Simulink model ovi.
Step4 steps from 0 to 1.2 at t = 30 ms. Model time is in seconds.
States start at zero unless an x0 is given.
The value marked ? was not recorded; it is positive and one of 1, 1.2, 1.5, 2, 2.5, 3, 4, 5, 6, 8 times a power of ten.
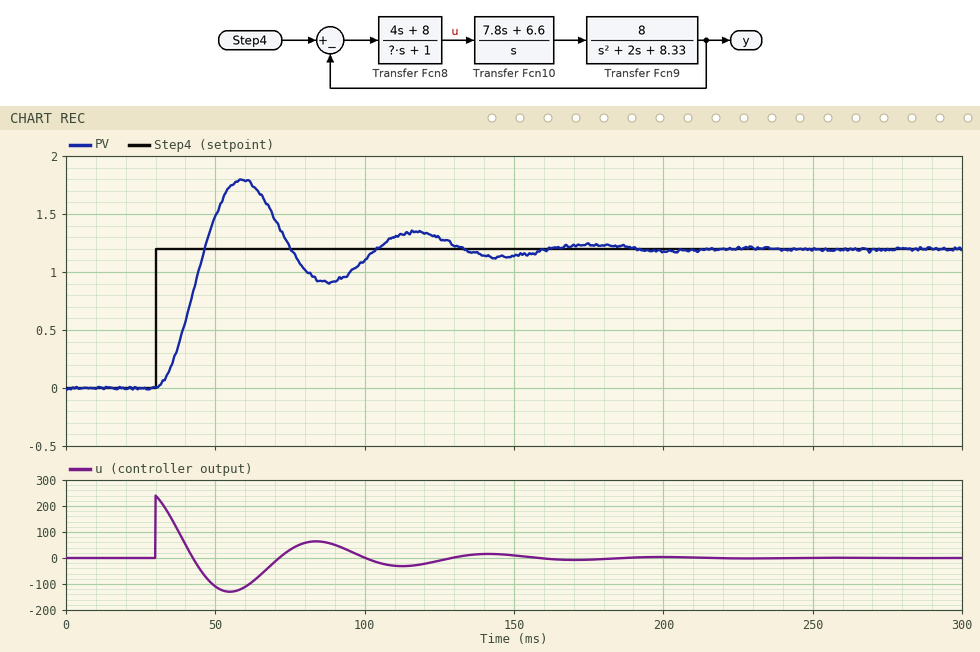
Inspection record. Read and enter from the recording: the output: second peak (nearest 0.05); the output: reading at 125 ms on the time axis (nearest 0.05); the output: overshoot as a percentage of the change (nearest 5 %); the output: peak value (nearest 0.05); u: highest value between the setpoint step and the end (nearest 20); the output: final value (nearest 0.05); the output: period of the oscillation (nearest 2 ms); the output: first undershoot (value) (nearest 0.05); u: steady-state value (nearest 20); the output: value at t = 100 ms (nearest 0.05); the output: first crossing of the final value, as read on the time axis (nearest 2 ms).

1.35
1.30
50 %
1.80
240
1.20
58 ms
0.90
0
1.10
46 ms
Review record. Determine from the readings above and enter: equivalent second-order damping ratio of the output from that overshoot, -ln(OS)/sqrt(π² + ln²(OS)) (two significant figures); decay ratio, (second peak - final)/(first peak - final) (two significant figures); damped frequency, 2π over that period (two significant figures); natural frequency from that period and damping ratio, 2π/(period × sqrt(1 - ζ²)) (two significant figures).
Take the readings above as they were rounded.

0.22
0.25
0.11 rad/ms
0.11 rad/ms
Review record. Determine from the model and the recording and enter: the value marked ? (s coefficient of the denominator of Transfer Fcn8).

0.02
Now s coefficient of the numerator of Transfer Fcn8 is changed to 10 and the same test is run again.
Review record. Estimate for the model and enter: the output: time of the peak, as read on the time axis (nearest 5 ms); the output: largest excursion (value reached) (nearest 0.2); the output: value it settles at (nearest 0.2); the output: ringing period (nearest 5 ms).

50 ms
2.0
1.2
35 ms
